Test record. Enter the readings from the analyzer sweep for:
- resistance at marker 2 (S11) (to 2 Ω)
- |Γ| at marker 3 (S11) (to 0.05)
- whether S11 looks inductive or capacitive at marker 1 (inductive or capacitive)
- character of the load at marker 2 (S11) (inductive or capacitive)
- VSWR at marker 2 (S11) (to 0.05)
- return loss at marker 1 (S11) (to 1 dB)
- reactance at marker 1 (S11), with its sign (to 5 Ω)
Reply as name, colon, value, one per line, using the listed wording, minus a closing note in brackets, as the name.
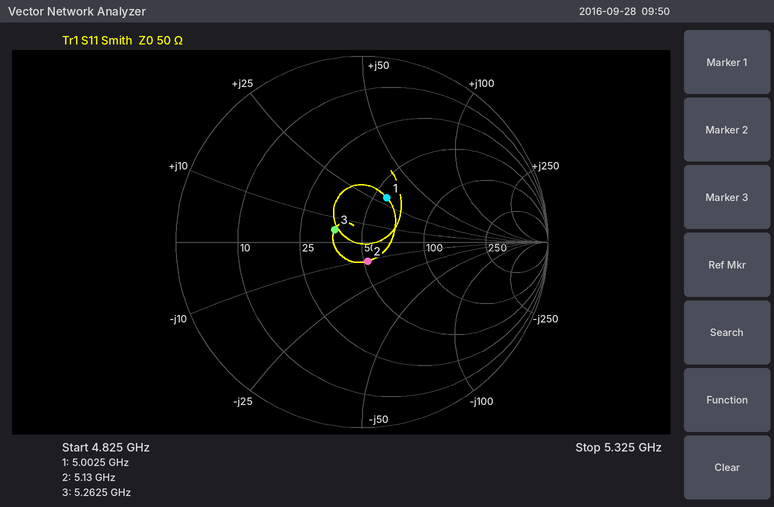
resistance at marker 2 (S11): 52 Ω
|Γ| at marker 3 (S11): 0.15
whether S11 looks inductive or capacitive at marker 1: inductive
character of the load at marker 2 (S11): capacitive
VSWR at marker 2 (S11): 1.25
return loss at marker 1 (S11): 11 dB
reactance at marker 1 (S11), with its sign: +30 Ω
